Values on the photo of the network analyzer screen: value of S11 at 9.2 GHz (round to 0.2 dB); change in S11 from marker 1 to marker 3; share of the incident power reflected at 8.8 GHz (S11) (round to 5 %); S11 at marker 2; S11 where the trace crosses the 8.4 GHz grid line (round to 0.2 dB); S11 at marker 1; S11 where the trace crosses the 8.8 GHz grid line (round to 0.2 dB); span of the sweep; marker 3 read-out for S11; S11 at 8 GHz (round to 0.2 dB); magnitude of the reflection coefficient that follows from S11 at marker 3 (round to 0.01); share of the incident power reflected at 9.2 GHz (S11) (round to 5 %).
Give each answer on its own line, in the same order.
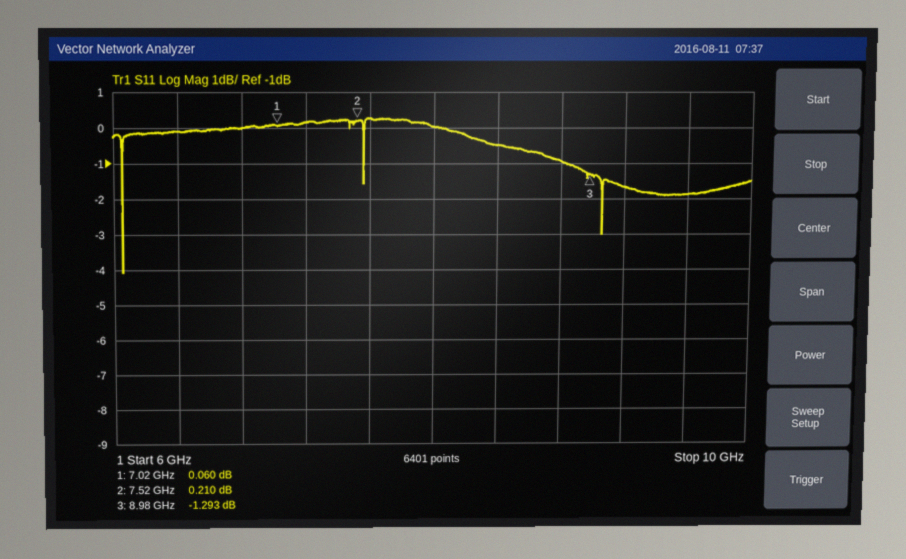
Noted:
-1.6 dB
-1.353 dB
80 %
0.210 dB
-0.4 dB
0.060 dB
-1.0 dB
4 GHz
-1.293 dB
0.0 dB
0.86
70 %
